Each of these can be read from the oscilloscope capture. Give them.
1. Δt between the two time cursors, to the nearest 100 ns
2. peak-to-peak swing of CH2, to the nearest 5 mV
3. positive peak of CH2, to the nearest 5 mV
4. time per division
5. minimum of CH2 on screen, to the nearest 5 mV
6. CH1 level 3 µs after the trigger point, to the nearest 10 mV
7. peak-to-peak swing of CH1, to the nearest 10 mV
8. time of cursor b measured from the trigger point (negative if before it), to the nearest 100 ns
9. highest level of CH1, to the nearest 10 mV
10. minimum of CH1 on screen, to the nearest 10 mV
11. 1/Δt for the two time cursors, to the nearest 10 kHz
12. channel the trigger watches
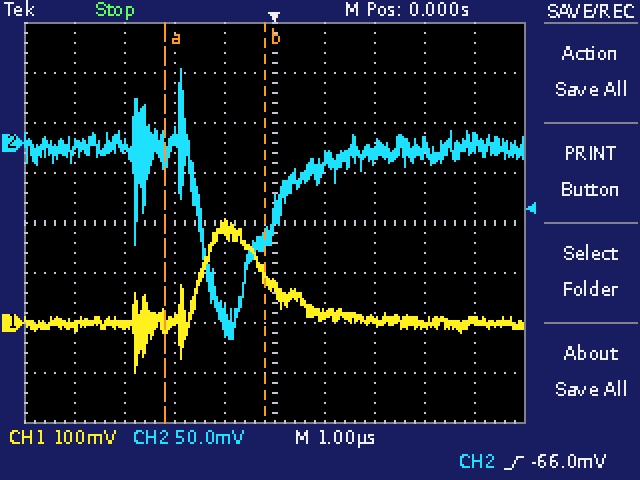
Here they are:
2.0 µs
270 mV
75 mV
1 µs
-195 mV
0 mV
310 mV
-200 ns
210 mV
-100 mV
500 kHz
CH2
